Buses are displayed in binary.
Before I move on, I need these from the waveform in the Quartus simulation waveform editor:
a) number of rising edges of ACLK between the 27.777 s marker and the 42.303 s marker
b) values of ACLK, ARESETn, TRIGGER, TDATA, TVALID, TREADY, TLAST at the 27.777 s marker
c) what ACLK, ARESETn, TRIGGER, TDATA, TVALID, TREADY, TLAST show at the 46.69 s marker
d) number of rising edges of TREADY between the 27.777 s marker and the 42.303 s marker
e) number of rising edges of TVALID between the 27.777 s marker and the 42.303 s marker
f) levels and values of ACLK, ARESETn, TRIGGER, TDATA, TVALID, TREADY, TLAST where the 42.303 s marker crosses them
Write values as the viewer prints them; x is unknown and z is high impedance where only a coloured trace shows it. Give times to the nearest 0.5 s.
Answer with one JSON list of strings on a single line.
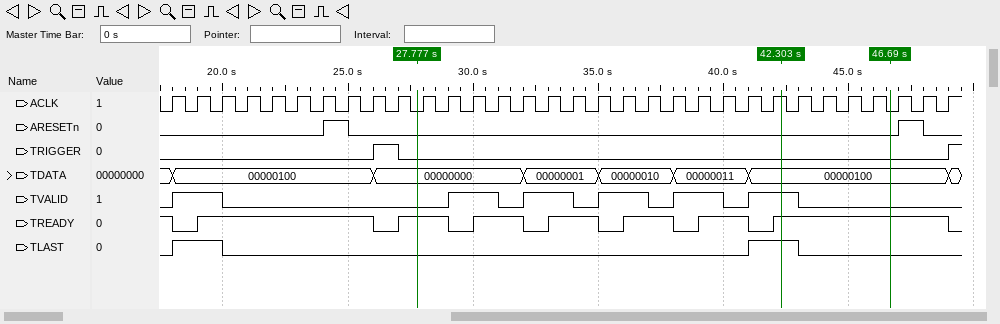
["15", "ACLK=0, ARESETn=0, TRIGGER=0, TDATA=00000000, TVALID=0, TREADY=1, TLAST=0", "ACLK=0, ARESETn=0, TRIGGER=0, TDATA=00000100, TVALID=0, TREADY=1, TLAST=0", "5", "5", "ACLK=1, ARESETn=0, TRIGGER=0, TDATA=00000100, TVALID=1, TREADY=1, TLAST=1"]
